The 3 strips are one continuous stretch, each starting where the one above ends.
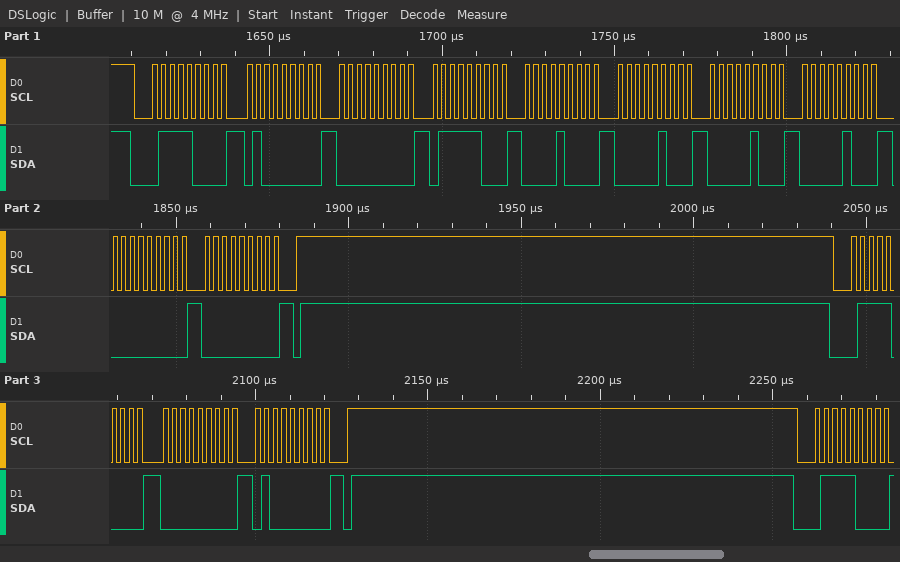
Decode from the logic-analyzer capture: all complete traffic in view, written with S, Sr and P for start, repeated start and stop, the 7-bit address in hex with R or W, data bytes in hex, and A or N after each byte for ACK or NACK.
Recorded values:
S 3CW A 40 A 00 A 7C A 08 A 04 A 04 A 04 A 00 A 00 A P S 3CW A 00 A 40 A P S 3CW A
